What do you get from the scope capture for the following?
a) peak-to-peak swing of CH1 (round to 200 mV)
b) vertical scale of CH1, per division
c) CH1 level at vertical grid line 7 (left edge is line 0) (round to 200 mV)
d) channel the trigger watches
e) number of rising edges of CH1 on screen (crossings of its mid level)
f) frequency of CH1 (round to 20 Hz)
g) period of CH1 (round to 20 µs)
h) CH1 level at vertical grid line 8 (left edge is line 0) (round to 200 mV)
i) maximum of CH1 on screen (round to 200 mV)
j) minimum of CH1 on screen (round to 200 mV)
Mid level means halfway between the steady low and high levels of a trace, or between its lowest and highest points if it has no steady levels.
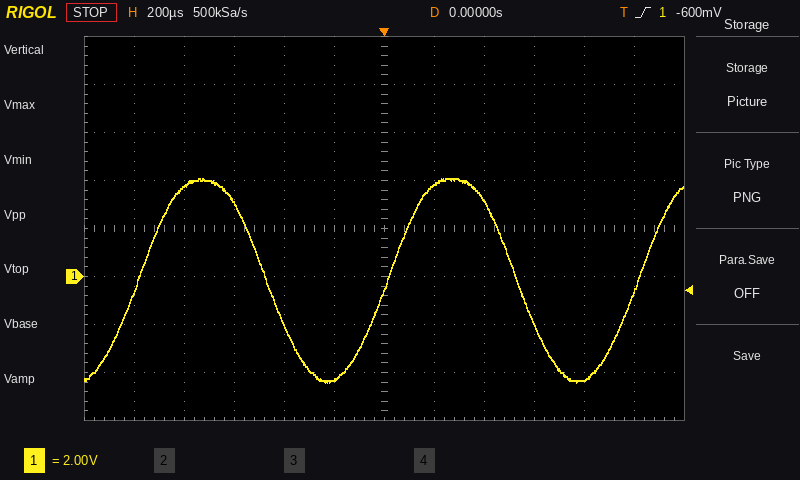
8.4 V
2 V
3.8 V
CH1
3
1.00 kHz
1.00 ms
3.2 V
4.0 V
-4.4 V
